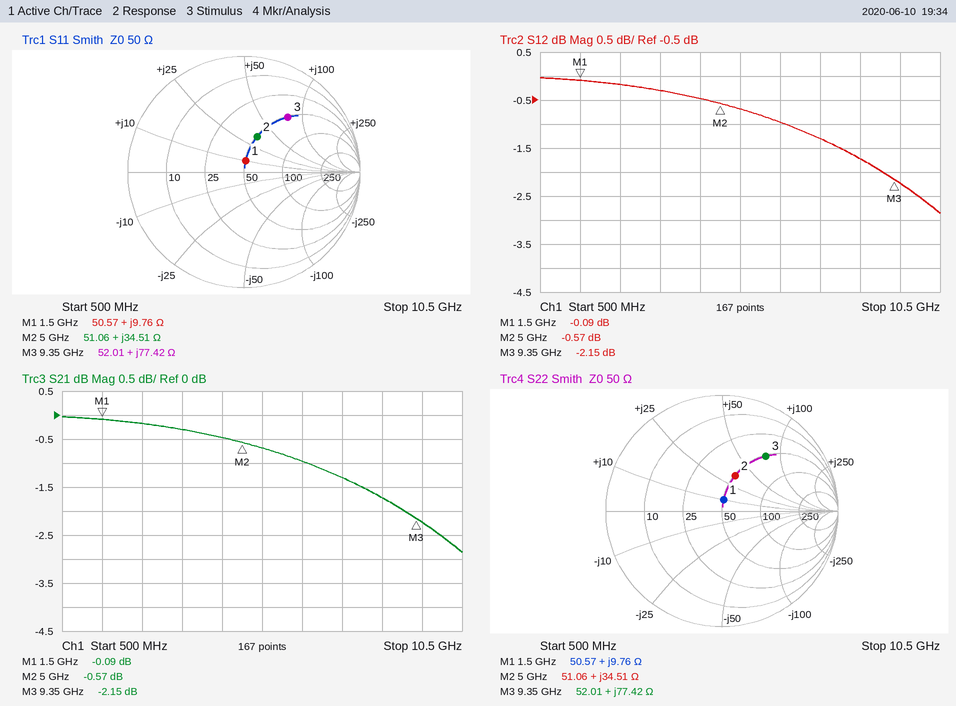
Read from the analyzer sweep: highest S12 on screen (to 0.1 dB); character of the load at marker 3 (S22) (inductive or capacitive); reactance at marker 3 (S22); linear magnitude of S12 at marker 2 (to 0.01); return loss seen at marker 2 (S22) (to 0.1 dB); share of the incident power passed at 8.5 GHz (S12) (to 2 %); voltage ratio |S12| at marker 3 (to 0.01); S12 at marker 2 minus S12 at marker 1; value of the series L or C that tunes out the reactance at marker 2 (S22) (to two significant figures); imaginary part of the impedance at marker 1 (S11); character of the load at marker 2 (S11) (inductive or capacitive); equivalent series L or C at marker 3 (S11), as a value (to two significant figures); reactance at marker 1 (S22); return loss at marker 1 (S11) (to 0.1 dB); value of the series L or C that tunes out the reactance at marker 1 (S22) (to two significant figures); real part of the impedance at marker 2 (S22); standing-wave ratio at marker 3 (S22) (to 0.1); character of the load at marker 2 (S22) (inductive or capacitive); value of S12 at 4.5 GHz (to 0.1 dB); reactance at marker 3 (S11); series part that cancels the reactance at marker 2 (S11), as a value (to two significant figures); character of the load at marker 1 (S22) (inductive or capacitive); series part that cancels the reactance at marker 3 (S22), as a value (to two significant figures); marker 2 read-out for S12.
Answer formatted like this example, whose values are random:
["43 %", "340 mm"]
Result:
["0.0 dB", "inductive", "+77.42 Ω", "0.94", "9.8 dB", "68 %", "0.78", "-0.48 dB", "920 fF", "+9.76 Ω", "inductive", "1.3 nH", "+9.76 Ω", "20.3 dB", "11 pF", "51.06 Ω", "4.1", "inductive", "-0.5 dB", "+77.42 Ω", "920 fF", "inductive", "220 fF", "-0.57 dB"]
